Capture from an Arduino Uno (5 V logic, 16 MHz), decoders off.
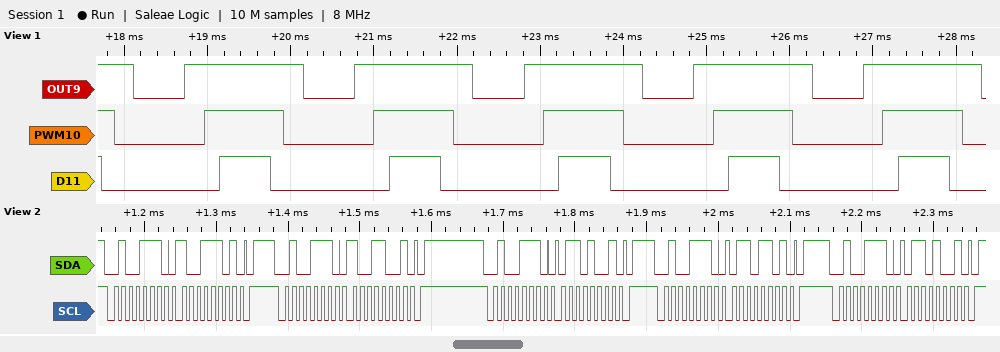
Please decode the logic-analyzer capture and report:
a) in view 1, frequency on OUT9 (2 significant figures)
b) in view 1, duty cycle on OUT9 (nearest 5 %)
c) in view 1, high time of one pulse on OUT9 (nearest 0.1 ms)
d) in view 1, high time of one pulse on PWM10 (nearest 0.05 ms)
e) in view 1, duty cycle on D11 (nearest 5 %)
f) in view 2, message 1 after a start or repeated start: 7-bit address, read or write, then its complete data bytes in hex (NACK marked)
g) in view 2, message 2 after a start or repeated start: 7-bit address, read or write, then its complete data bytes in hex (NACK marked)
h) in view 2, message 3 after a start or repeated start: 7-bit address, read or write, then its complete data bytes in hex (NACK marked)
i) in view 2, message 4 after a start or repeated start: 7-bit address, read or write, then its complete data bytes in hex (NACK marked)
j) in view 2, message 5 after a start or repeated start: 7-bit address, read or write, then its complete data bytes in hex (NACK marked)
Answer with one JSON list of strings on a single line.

["490 Hz", "70 %", "1.4 ms", "0.95 ms", "30 %", "0x27 write: 9D", "0x27 write: 99", "0x27 write: 69", "0x27 write: 6D", "0x27 write: 69"]
